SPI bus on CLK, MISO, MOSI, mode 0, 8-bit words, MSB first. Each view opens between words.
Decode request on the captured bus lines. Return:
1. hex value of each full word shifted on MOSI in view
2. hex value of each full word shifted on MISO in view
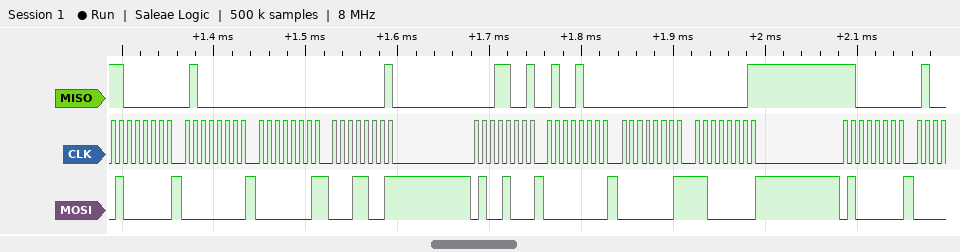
40, 00, 01, 19, 48, 00, 01, C0, 40
C0, 40, 00, 01, 19, 48, 00, 01, C0
